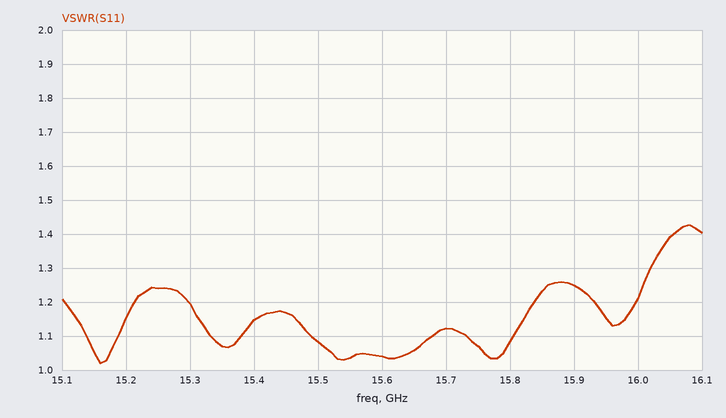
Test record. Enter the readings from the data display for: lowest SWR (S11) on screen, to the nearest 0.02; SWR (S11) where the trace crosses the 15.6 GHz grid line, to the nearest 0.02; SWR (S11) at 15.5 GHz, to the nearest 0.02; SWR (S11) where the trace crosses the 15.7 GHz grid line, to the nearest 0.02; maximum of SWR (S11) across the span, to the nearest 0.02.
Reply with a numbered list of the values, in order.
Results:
1. 1.02
2. 1.04
3. 1.08
4. 1.12
5. 1.42
